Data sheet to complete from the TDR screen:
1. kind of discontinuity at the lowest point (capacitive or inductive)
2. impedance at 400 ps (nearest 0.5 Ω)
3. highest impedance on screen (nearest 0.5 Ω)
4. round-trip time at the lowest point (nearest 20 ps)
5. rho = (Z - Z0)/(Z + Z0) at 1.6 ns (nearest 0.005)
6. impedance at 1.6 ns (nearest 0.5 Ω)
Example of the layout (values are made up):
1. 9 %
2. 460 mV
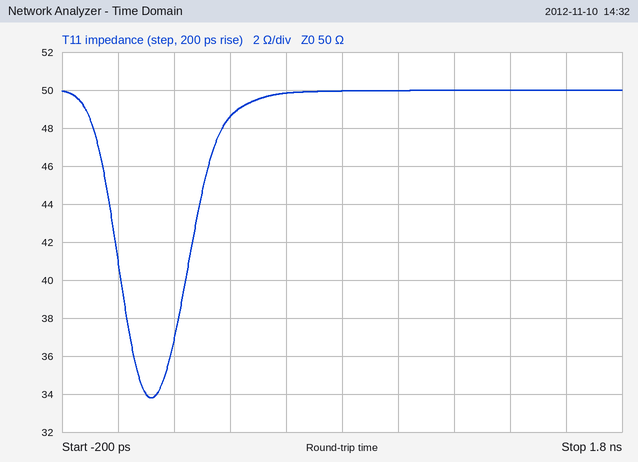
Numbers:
1. capacitive
2. 48.5 Ω
3. 50.0 Ω
4. 120 ps
5. 0.000
6. 50.0 Ω
